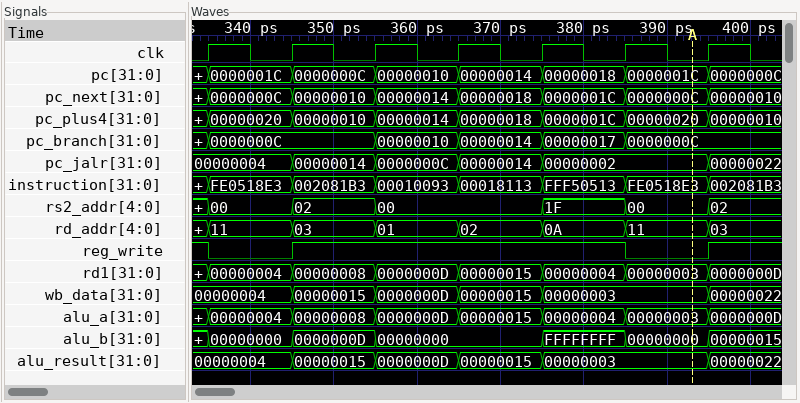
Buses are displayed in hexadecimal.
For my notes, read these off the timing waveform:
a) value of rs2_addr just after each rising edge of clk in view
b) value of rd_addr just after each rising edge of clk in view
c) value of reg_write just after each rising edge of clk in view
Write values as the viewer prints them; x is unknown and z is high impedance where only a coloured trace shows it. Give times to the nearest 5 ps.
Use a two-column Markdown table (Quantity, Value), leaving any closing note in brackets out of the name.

| Quantity | Value |
|---|---|
| value of rs2_addr just after each rising edge of clk in view | 00, 02, 00, 00, 1F, 00, 02 |
| value of rd_addr just after each rising edge of clk in view | 11, 03, 01, 02, 0A, 11, 03 |
| value of reg_write just after each rising edge of clk in view | 0 1 1 1 1 0 1 |
